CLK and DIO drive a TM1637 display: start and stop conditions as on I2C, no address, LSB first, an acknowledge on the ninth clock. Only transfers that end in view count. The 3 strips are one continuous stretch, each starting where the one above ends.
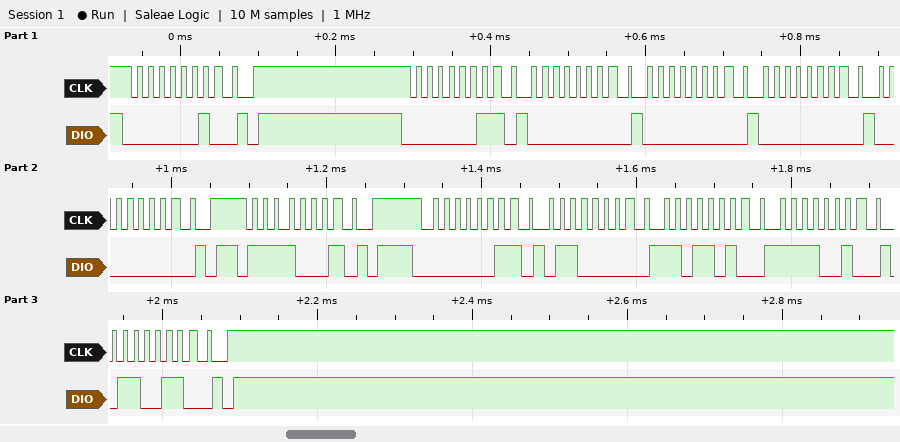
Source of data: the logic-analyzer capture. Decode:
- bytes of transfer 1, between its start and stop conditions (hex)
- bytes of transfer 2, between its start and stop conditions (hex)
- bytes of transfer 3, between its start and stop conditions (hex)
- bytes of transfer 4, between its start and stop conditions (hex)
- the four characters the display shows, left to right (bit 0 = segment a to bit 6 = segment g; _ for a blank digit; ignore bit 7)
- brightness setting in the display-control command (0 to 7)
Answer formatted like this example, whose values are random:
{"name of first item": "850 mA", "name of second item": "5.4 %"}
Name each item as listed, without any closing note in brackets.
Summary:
{"bytes of transfer 1, between its start and stop conditions": "40", "bytes of transfer 2, between its start and stop conditions": "C0 00 00 00 00", "bytes of transfer 3, between its start and stop conditions": "8F", "bytes of transfer 4, between its start and stop conditions": "C0 06 5B 4F 66", "the four characters the display shows, left to right": "1234", "brightness setting in the display-control command": "7"}
